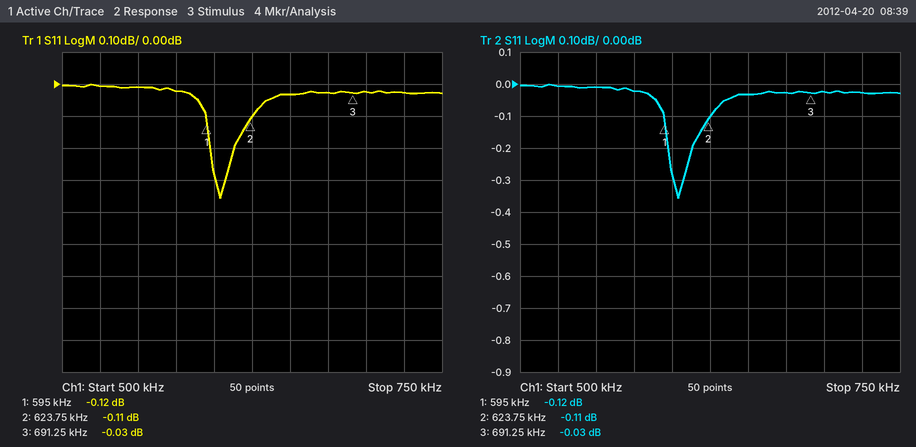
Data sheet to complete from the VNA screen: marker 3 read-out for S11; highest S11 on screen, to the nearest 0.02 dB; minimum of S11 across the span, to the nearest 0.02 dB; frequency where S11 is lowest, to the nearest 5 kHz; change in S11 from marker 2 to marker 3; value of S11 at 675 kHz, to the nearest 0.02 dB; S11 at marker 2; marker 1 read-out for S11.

-0.03 dB
0.00 dB
-0.36 dB
605 kHz
0.08 dB
-0.02 dB
-0.11 dB
-0.12 dB
